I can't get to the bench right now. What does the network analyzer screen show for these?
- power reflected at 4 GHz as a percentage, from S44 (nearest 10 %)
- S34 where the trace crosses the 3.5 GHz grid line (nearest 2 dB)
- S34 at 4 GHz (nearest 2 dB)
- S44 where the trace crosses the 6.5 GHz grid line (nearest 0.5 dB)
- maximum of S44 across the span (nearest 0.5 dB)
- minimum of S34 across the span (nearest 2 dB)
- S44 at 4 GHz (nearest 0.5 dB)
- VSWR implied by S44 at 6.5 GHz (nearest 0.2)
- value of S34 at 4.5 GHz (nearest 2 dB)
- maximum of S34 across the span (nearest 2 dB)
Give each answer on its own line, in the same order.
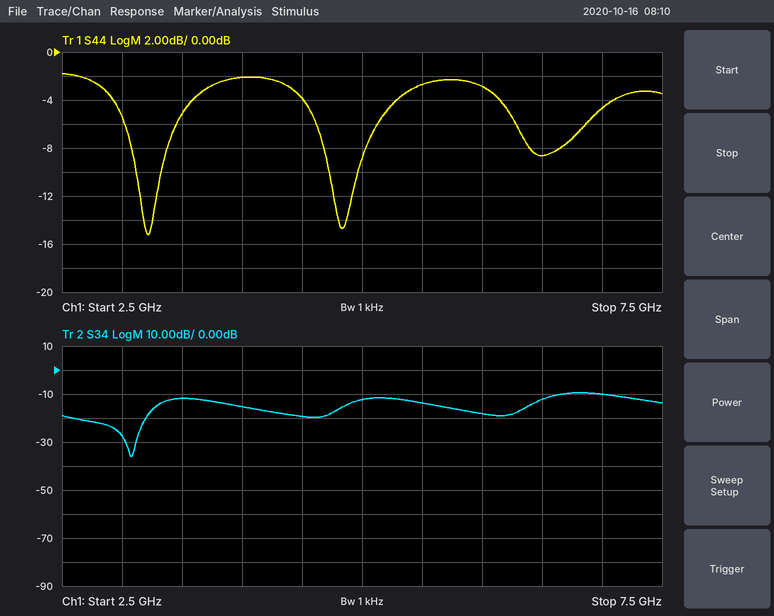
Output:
60 %
-12 dB
-16 dB
-8.5 dB
-2.0 dB
-36 dB
-2.0 dB
2.2
-20 dB
-10 dB
